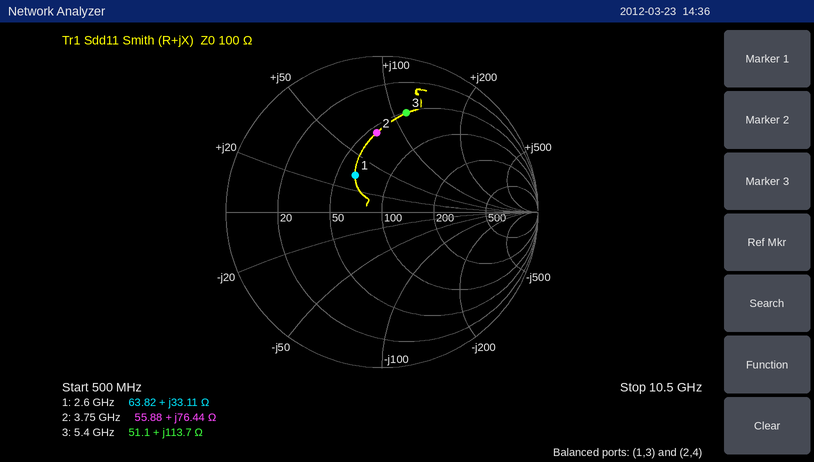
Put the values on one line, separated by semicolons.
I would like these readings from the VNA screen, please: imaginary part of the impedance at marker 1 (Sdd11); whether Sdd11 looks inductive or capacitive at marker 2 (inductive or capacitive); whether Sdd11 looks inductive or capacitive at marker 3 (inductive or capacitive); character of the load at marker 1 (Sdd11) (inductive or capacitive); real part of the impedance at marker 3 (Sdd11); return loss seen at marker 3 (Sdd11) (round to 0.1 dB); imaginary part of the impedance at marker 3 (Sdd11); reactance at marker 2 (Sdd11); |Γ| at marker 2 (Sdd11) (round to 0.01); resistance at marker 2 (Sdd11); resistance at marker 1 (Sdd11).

+33.11 Ω; inductive; inductive; inductive; 51.1 Ω; 3.7 dB; +113.7 Ω; +76.44 Ω; 0.51; 55.88 Ω; 63.82 Ω
